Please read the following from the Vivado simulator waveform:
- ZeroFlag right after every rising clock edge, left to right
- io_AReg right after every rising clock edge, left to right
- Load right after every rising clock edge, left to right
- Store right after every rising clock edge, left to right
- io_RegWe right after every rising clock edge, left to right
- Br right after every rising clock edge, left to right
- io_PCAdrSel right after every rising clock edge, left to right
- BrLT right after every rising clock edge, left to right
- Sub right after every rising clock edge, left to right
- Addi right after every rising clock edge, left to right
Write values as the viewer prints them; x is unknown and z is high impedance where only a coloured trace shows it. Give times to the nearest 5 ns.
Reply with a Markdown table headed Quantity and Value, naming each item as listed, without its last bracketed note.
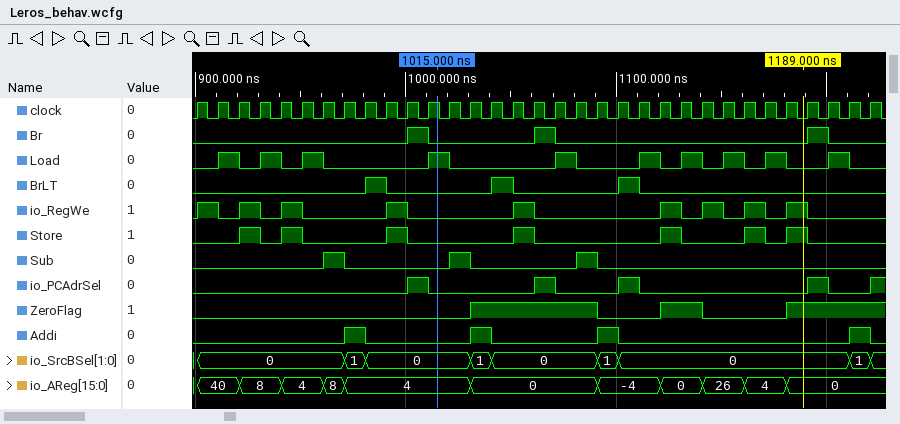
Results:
| Quantity | Value |
|---|---|
| ZeroFlag right after every rising clock edge, left to right | 0 0 0 0 0 0 0 0 0 0 0 0 0 1 1 1 1 1 1 0 0 0 1 1 0 0 0 0 1 1 1 1 1 |
| io_AReg right after every rising clock edge, left to right | 40, 40, 8, 8, 4, 4, 8, 4, 4, 4, 4, 4, 4, 0, 0, 0, 0, 0, 0, -4, -4, -4, 0, 0, 26, 26, 4, 4, 0, 0, 0, 0, 0 |
| Load right after every rising clock edge, left to right | 0 1 0 1 0 1 0 0 0 0 0 1 0 0 0 0 0 1 0 0 0 1 0 1 0 1 0 1 0 0 1 0 0 |
| Store right after every rising clock edge, left to right | 0 0 1 0 1 0 0 0 0 1 0 0 0 0 0 1 0 0 0 0 0 0 1 0 0 0 1 0 1 0 0 0 0 |
| io_RegWe right after every rising clock edge, left to right | 1 0 1 0 1 0 0 0 0 1 0 0 0 0 0 1 0 0 0 0 0 0 1 0 1 0 1 0 1 0 0 0 0 |
| Br right after every rising clock edge, left to right | 0 0 0 0 0 0 0 0 0 0 1 0 0 0 0 0 1 0 0 0 0 0 0 0 0 0 0 0 0 1 0 0 0 |
| io_PCAdrSel right after every rising clock edge, left to right | 0 0 0 0 0 0 0 0 0 0 1 0 0 0 0 0 1 0 0 0 1 0 0 0 0 0 0 0 0 1 0 0 1 |
| BrLT right after every rising clock edge, left to right | 0 0 0 0 0 0 0 0 1 0 0 0 0 0 1 0 0 0 0 0 1 0 0 0 0 0 0 0 0 0 0 0 0 |
| Sub right after every rising clock edge, left to right | 0 0 0 0 0 0 1 0 0 0 0 0 1 0 0 0 0 0 1 0 0 0 0 0 0 0 0 0 0 0 0 0 0 |
| Addi right after every rising clock edge, left to right | 0 0 0 0 0 0 0 1 0 0 0 0 0 1 0 0 0 0 0 1 0 0 0 0 0 0 0 0 0 0 0 1 0 |
